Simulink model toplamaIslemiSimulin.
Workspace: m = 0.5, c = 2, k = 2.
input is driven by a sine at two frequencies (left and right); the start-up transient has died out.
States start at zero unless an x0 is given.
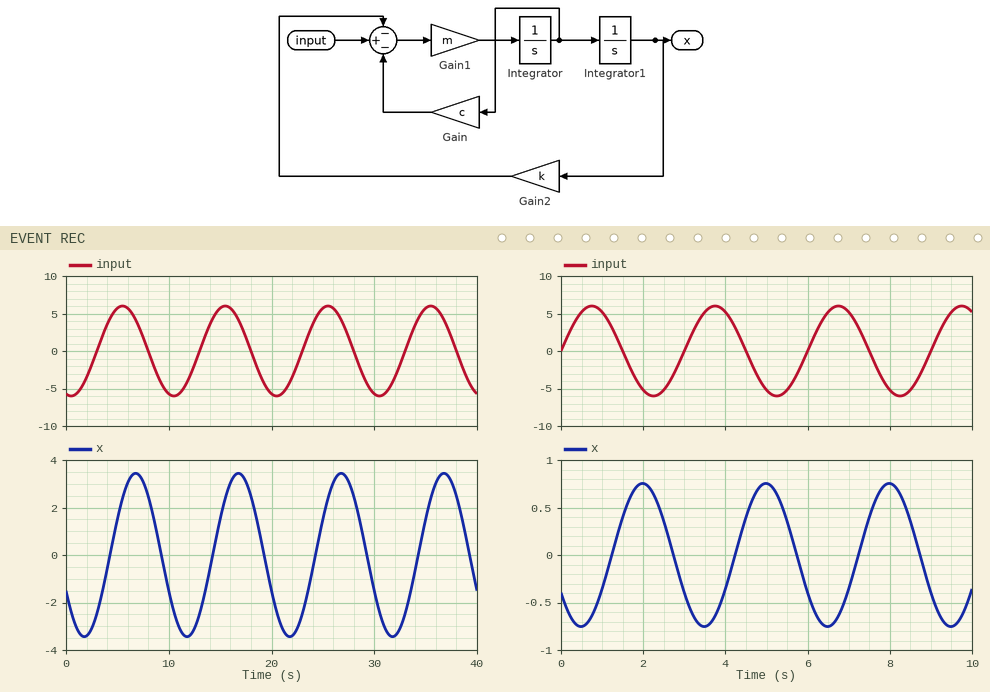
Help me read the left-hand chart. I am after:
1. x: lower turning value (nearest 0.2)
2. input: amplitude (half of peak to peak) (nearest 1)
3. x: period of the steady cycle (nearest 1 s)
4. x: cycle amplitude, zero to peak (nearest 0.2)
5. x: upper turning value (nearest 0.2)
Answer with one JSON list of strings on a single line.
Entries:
["-3.4", "6", "10 s", "3.4", "3.4"]
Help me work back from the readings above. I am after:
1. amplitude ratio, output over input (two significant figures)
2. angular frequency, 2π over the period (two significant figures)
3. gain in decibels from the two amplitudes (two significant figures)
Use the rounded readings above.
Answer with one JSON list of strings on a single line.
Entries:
["0.57", "0.63 rad/s", "-4.9 dB"]
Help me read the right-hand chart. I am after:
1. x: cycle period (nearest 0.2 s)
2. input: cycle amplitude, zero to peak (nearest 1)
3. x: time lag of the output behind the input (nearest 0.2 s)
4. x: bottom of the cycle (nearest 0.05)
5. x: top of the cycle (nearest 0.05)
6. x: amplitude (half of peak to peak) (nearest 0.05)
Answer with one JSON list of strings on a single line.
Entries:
["3.0 s", "6", "1.2 s", "-0.75", "0.75", "0.75"]
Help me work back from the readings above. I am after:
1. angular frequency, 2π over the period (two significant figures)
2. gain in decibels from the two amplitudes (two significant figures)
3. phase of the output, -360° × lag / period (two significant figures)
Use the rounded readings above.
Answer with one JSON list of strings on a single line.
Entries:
["2.1 rad/s", "-18 dB", "-140°"]
